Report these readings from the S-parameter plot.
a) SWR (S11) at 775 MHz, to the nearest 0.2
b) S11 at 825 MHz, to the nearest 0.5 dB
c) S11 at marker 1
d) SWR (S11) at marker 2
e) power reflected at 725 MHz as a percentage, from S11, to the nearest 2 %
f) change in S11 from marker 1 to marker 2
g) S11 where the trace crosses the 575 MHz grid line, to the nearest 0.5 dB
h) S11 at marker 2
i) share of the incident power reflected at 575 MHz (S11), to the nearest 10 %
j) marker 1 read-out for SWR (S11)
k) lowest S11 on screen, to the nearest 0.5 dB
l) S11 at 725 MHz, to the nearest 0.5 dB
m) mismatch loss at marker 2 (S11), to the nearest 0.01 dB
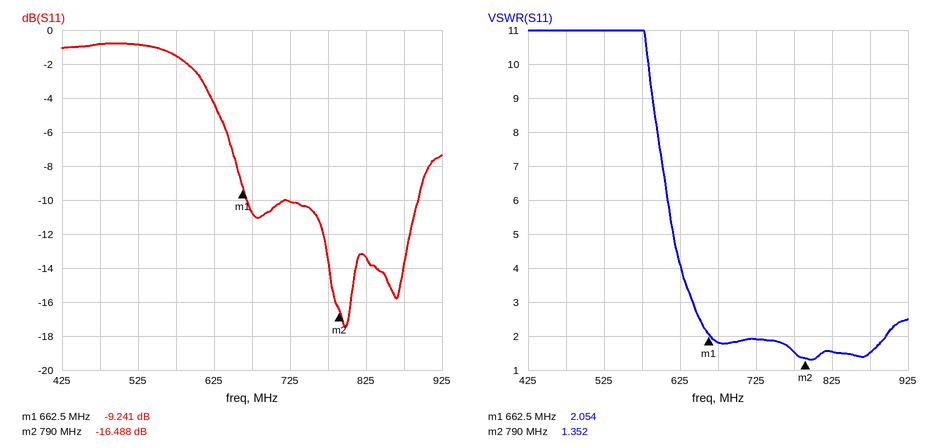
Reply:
1.6
-13.5 dB
-9.241 dB
1.352
10 %
-7.247 dB
-1.5 dB
-16.488 dB
70 %
2.054
-17.5 dB
-10.0 dB
0.10 dB
